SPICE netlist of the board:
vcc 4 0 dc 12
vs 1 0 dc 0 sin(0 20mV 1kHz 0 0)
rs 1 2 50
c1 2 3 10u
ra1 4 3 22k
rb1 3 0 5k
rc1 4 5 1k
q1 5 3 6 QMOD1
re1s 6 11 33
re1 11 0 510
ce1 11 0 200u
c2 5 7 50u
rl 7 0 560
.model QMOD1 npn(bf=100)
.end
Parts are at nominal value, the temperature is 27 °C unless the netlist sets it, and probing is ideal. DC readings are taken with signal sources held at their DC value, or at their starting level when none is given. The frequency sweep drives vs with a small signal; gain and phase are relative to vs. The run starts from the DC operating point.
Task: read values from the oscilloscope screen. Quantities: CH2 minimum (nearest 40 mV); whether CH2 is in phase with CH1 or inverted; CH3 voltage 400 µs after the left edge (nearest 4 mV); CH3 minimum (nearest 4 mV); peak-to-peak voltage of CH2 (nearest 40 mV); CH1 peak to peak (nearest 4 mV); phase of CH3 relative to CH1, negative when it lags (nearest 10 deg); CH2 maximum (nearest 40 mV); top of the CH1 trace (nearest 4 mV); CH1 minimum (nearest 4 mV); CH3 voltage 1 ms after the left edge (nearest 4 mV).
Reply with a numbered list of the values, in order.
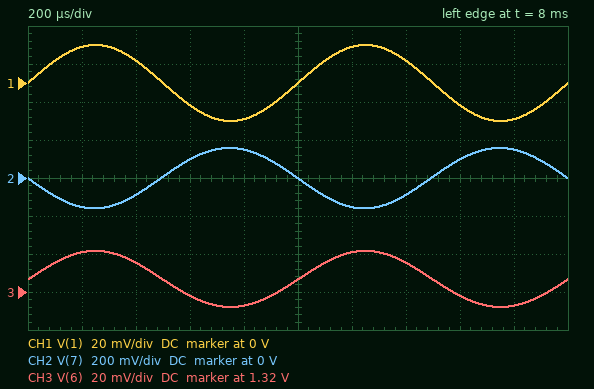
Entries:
1. -160 mV
2. inverted
3. 1.336 V
4. 1.312 V
5. 320 mV
6. 40 mV
7. 0 deg
8. 160 mV
9. 20 mV
10. -20 mV
11. 1.328 V
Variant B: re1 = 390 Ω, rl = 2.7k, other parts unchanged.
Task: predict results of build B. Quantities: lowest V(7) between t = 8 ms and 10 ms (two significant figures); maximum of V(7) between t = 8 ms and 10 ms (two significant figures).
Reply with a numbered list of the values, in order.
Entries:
1. -340 mV
2. 340 mV
